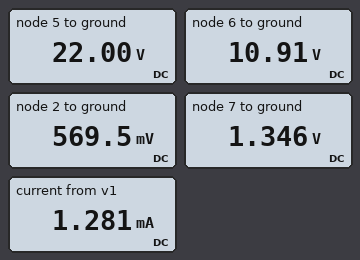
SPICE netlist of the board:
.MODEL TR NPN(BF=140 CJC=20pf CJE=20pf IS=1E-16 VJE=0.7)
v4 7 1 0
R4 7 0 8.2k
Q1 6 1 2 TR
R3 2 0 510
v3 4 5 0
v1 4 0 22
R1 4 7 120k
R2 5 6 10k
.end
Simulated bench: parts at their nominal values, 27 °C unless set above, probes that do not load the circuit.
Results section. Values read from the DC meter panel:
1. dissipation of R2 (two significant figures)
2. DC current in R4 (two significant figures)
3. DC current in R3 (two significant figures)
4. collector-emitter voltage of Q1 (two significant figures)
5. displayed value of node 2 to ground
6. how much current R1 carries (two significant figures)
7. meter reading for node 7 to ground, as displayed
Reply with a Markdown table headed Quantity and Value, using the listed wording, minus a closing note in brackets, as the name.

| Quantity | Value |
|---|---|
| dissipation of R2 | 12 mW |
| DC current in R4 | 160 µA |
| DC current in R3 | 1.1 mA |
| collector-emitter voltage of Q1 | 10 V |
| displayed value of node 2 to ground | 569.5 mV |
| how much current R1 carries | 170 µA |
| meter reading for node 7 to ground, as displayed | 1.346 V |
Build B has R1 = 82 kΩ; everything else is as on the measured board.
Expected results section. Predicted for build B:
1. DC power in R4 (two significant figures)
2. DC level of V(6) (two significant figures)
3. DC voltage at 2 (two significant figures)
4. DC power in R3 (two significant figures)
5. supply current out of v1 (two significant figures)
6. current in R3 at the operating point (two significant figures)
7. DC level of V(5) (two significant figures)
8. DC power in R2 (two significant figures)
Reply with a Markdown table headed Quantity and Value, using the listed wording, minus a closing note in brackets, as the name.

| Quantity | Value |
|---|---|
| DC power in R4 | 420 µW |
| DC level of V(6) | 1.2 V |
| DC voltage at 2 | 1.1 V |
| DC power in R3 | 2.2 mW |
| supply current out of v1 | 2.3 mA |
| current in R3 at the operating point | 2.1 mA |
| DC level of V(5) | 22 V |
| DC power in R2 | 43 mW |
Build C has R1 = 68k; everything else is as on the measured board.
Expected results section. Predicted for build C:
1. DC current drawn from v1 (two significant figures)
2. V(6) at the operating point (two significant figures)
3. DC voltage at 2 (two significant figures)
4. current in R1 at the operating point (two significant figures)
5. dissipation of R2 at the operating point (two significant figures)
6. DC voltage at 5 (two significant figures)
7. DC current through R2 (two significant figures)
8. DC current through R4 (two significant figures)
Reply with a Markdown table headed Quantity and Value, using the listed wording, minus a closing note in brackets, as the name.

| Quantity | Value |
|---|---|
| DC current drawn from v1 | 2.4 mA |
| V(6) at the operating point | 1.2 V |
| DC voltage at 2 | 1.1 V |
| current in R1 at the operating point | 300 µA |
| dissipation of R2 at the operating point | 43 mW |
| DC voltage at 5 | 22 V |
| DC current through R2 | 2.1 mA |
| DC current through R4 | 230 µA |
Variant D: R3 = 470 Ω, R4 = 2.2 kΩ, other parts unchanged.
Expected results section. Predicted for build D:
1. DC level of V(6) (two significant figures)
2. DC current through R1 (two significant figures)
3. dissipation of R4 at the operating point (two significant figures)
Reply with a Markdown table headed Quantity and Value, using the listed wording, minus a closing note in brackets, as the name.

| Quantity | Value |
|---|---|
| DC level of V(6) | 22 V |
| DC current through R1 | 180 µA |
| dissipation of R4 at the operating point | 71 µW |
